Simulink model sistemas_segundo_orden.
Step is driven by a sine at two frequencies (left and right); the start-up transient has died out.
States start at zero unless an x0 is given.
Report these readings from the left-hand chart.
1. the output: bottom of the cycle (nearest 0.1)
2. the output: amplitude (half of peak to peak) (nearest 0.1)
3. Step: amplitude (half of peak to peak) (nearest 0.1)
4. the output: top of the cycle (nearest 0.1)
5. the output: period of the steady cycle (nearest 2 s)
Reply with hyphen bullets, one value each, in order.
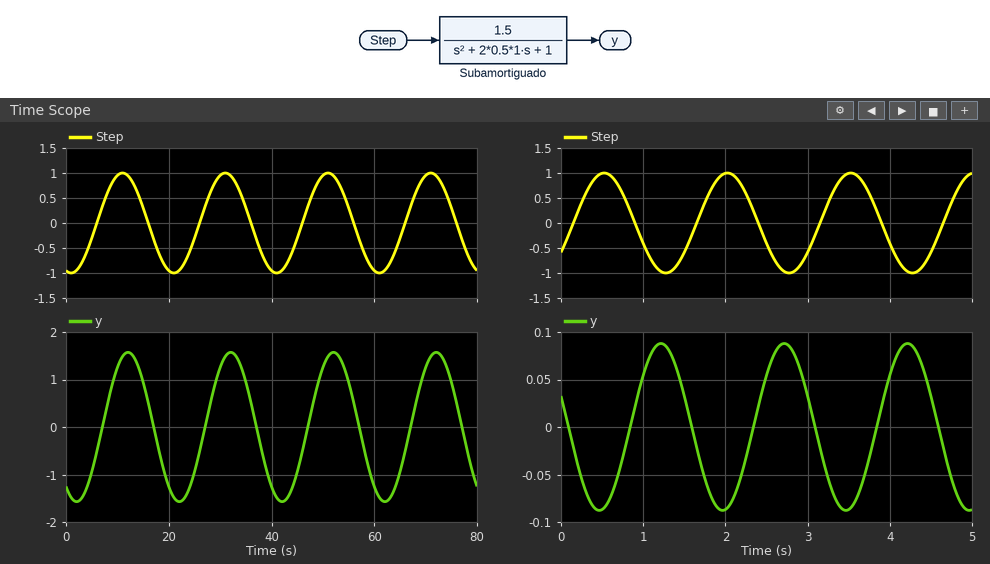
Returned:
- -1.6
- 1.6
- 1.0
- 1.6
- 20 s
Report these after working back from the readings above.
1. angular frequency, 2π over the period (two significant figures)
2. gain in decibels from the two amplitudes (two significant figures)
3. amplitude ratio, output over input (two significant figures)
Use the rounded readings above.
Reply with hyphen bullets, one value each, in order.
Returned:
- 0.31 rad/s
- 4.1 dB
- 1.6
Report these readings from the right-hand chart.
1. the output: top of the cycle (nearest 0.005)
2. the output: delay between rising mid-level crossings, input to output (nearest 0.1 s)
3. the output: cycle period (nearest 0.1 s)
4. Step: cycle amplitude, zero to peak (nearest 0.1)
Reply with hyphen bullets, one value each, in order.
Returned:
- 0.090
- 0.7 s
- 1.5 s
- 1.0
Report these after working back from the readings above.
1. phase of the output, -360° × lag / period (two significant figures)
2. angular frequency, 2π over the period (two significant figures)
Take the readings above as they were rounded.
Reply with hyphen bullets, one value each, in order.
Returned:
- -170°
- 4.2 rad/s
